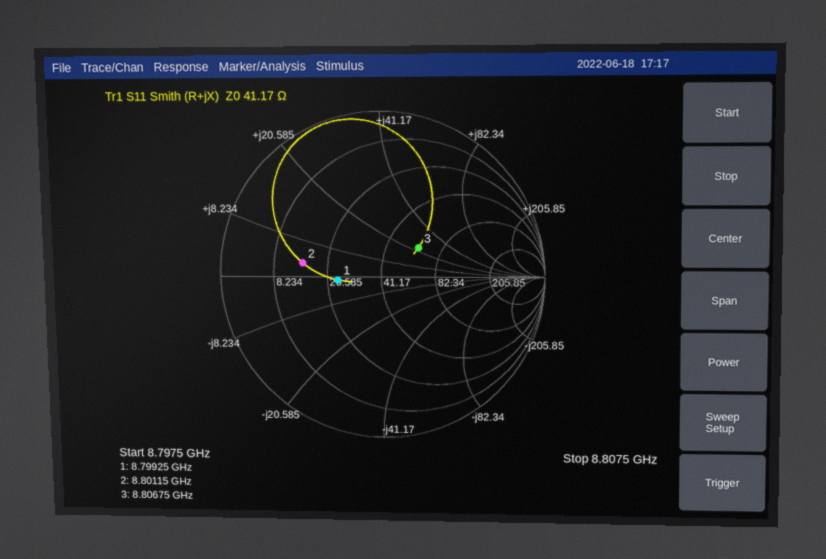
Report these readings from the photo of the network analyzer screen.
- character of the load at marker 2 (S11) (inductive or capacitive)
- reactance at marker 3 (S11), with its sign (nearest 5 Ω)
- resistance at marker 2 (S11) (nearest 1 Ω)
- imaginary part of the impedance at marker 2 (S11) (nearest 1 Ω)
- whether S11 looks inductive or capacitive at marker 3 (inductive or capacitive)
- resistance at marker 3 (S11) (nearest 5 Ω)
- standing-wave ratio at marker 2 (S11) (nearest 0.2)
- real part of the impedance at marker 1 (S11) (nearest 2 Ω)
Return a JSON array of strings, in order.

["inductive", "+25 Ω", "14 Ω", "+3 Ω", "inductive", "60 Ω", "3.0", "24 Ω"]
